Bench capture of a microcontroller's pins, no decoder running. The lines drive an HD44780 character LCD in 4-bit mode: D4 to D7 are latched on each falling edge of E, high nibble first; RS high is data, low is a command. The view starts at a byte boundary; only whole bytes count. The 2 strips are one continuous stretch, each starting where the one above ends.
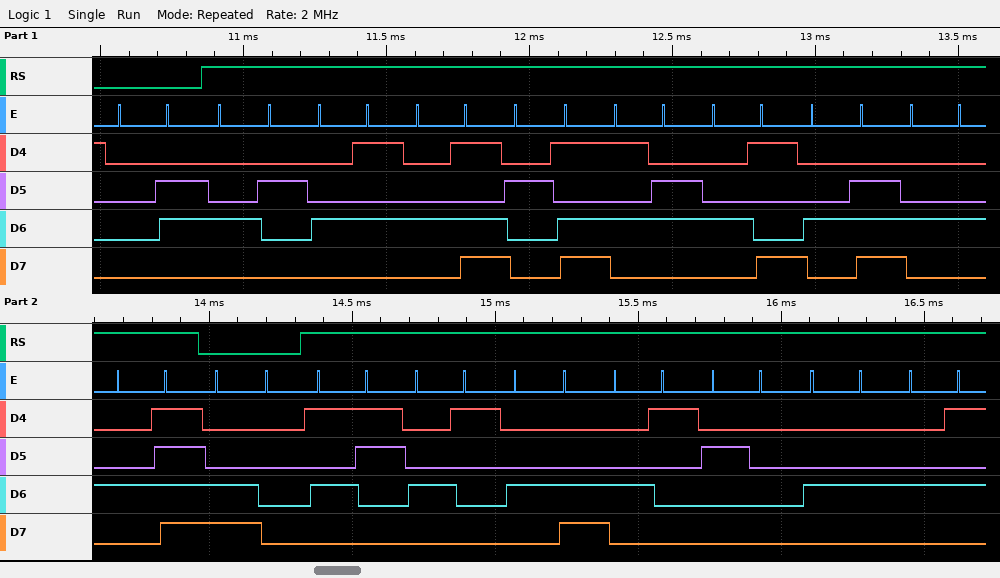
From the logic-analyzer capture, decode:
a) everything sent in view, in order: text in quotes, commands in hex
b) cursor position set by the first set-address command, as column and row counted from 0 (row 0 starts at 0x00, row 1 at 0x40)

0x06 "BEM-VINDO" 0xC0 "SALA DE"
column 0, row 1
